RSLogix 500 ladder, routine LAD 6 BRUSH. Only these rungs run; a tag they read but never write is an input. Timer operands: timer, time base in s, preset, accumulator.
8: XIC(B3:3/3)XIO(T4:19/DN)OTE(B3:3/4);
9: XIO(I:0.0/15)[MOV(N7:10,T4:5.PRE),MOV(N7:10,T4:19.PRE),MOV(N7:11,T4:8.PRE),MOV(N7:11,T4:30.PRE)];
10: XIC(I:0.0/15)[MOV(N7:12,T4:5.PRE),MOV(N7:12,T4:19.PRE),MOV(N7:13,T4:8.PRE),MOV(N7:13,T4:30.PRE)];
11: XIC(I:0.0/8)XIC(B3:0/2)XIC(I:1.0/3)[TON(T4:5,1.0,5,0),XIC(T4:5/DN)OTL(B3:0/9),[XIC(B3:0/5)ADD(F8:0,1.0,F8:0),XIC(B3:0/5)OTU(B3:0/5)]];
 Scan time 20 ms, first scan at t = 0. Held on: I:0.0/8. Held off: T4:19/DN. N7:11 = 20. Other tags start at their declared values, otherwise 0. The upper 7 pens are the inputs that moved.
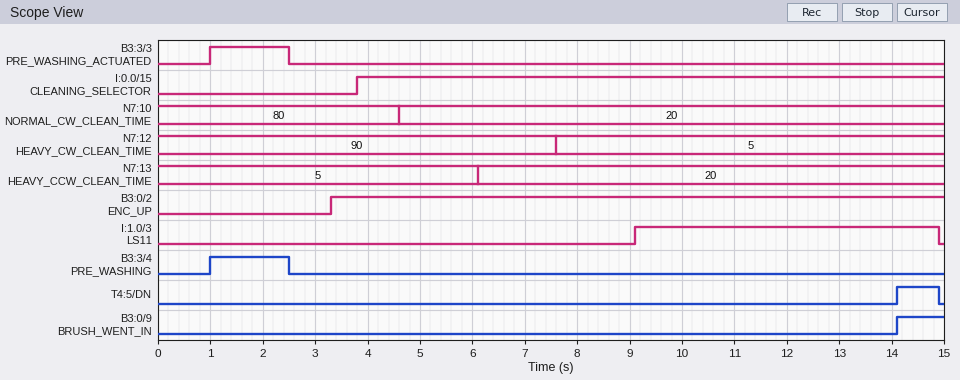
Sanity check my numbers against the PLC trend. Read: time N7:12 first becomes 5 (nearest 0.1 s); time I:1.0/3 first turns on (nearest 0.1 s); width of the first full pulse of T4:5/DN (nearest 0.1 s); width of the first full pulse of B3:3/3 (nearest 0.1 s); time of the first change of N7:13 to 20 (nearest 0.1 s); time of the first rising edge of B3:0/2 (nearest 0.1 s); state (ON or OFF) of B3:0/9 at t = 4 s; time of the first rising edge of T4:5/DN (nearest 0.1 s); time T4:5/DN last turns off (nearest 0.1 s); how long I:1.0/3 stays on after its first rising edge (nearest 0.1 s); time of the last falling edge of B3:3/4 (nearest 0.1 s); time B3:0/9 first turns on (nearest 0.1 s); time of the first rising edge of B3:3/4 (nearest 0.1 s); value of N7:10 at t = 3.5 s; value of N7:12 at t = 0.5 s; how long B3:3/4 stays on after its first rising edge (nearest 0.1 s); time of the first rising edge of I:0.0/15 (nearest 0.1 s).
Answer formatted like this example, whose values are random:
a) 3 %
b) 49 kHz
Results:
a) 7.6 s
b) 9.1 s
c) 0.8 s
d) 1.5 s
e) 6.1 s
f) 3.3 s
g) OFF
h) 14.1 s
i) 14.9 s
j) 5.8 s
k) 2.5 s
l) 14.1 s
m) 1.0 s
n) 80
o) 90
p) 1.5 s
q) 3.8 s
